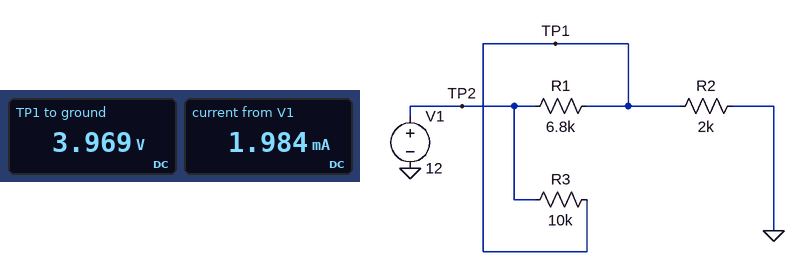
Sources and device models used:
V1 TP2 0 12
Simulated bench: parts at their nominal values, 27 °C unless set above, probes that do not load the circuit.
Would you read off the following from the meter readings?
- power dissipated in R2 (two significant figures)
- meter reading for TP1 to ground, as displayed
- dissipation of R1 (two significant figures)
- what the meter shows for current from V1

7.9 mW
3.969 V
9.5 mW
1.984 mA
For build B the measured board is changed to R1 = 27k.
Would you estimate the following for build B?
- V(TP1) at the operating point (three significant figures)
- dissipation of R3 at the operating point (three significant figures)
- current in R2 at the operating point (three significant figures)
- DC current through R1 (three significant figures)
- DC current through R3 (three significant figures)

2.58 V
8.87 mW
1.29 mA
349 µA
942 µA
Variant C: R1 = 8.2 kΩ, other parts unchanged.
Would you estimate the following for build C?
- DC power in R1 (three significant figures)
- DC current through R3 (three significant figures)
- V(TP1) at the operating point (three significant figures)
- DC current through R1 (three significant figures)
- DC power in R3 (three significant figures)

8.42 mW
831 µA
3.69 V
1.01 mA
6.91 mW
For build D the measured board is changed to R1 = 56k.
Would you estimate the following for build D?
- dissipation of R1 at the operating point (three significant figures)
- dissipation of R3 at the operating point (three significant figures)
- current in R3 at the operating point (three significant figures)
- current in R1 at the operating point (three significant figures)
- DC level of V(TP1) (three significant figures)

1.68 mW
9.43 mW
971 µA
173 µA
2.29 V
